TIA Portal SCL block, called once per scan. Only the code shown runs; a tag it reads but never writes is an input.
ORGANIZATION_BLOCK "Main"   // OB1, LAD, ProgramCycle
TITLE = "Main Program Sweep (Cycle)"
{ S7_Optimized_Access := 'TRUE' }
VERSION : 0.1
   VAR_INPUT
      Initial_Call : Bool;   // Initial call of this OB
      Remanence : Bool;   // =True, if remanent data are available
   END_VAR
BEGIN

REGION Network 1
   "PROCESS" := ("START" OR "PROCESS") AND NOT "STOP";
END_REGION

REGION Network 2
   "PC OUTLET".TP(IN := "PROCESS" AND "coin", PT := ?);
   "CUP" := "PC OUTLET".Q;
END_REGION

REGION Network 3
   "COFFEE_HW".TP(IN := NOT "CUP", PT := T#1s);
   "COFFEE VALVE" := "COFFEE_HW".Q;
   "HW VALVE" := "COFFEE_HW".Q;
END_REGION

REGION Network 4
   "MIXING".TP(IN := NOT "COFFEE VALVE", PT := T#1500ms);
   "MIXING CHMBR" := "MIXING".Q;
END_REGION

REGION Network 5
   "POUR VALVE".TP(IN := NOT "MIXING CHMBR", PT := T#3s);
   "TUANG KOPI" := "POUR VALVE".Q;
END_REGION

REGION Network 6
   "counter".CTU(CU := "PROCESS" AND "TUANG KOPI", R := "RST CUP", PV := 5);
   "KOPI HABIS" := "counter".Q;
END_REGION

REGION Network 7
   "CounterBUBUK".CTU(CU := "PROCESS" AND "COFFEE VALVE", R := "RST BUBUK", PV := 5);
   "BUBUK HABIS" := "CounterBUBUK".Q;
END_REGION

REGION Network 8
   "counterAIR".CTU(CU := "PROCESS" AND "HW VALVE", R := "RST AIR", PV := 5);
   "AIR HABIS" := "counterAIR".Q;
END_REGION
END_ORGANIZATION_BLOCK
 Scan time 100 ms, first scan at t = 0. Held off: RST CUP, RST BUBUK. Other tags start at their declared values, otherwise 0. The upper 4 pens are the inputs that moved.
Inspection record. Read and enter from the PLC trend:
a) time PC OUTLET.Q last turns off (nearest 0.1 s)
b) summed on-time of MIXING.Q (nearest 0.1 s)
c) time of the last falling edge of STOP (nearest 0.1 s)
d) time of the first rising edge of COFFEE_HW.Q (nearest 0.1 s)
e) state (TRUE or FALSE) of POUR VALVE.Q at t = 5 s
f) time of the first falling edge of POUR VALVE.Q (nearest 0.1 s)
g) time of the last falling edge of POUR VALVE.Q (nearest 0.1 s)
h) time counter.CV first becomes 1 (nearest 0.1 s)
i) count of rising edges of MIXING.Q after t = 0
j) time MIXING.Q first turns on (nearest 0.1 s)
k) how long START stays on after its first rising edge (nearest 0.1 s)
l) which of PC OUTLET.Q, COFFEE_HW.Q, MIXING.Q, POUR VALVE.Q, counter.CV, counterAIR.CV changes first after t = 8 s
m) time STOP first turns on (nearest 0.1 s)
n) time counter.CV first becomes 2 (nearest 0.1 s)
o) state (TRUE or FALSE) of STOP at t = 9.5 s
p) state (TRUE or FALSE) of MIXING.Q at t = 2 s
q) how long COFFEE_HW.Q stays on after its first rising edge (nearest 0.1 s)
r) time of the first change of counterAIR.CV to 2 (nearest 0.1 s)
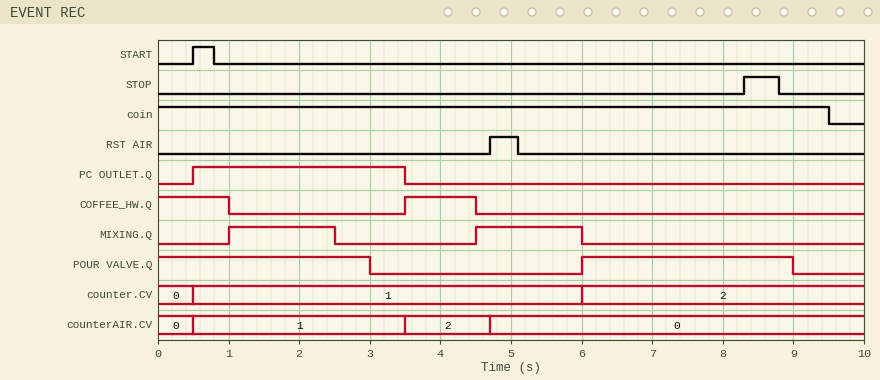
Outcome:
3.5 s
3.0 s
8.8 s
3.5 s
FALSE
3.0 s
9.0 s
0.5 s
2
1.0 s
0.3 s
POUR VALVE.Q
8.3 s
6.0 s
FALSE
TRUE
1.0 s
3.5 s
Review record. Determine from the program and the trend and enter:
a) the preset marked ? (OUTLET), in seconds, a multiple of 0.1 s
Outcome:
3.0 s
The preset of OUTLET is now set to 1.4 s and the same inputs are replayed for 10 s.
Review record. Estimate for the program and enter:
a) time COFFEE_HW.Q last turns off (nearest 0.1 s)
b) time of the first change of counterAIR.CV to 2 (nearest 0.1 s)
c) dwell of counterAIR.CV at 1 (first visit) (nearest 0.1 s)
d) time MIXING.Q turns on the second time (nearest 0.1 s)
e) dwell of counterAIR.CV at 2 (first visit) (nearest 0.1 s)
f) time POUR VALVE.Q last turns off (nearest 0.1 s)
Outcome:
2.9 s
1.9 s
1.4 s
2.9 s
2.8 s
7.4 s
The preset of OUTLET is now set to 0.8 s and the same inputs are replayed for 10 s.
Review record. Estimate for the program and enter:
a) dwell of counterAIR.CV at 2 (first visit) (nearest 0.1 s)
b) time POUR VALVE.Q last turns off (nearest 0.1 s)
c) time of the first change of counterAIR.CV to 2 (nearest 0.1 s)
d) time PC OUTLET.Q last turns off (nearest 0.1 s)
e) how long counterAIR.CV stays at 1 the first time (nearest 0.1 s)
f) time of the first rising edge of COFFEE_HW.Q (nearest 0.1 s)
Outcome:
3.4 s
3.0 s
1.3 s
1.3 s
0.8 s
1.3 s
